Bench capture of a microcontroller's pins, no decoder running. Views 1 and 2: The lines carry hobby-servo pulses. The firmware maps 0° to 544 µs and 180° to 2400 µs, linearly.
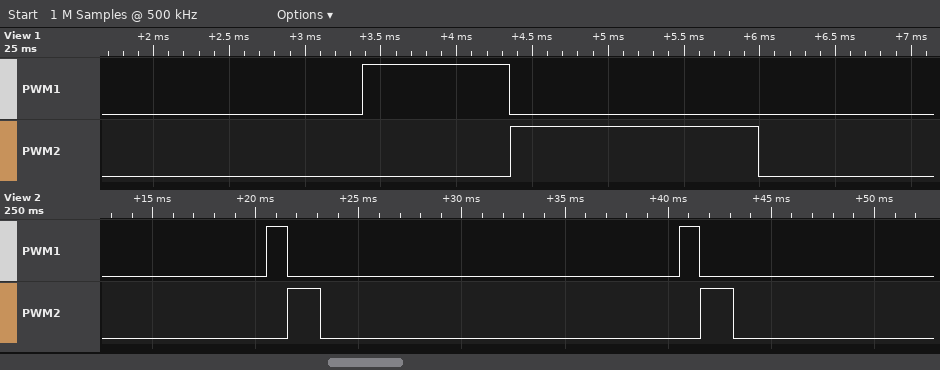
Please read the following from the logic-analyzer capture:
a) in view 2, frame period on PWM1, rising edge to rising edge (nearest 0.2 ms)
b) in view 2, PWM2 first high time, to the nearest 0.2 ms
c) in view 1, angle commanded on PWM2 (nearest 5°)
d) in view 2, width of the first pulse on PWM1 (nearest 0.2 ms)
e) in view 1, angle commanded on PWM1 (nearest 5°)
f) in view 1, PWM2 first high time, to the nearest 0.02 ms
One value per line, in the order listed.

20.0 ms
1.6 ms
105°
1.0 ms
40°
1.64 ms
